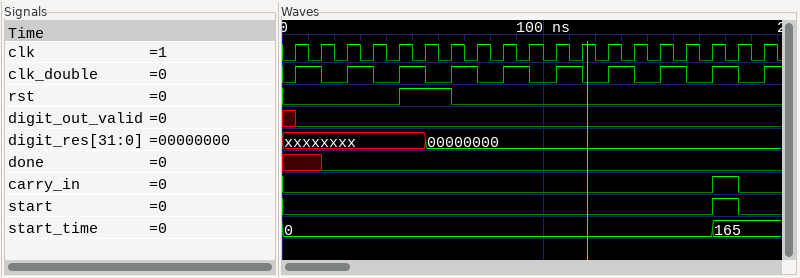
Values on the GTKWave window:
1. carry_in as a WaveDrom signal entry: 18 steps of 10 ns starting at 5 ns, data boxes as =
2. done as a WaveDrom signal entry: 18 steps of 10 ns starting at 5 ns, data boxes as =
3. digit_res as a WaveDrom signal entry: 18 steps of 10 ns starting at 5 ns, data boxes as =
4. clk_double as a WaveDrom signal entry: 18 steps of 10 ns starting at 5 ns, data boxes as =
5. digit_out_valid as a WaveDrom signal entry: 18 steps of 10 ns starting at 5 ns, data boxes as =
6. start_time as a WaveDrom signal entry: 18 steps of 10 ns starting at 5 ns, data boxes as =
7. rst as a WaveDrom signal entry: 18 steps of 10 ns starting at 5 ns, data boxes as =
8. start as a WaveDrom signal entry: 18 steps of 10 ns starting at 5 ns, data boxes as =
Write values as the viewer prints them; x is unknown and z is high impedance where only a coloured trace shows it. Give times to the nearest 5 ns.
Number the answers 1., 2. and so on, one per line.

1. {name: 'carry_in', wave: '0...............10'}
2. {name: 'done', wave: 'x0................'}
3. {name: 'digit_res', wave: 'x....=............', data: '00000000'}
4. {name: 'clk_double', wave: '101010101010101010'}
5. {name: 'digit_out_valid', wave: '0.................'}
6. {name: 'start_time', wave: '=...............=.', data: '0 165'}
7. {name: 'rst', wave: '0...1.0...........'}
8. {name: 'start', wave: '0...............10'}
